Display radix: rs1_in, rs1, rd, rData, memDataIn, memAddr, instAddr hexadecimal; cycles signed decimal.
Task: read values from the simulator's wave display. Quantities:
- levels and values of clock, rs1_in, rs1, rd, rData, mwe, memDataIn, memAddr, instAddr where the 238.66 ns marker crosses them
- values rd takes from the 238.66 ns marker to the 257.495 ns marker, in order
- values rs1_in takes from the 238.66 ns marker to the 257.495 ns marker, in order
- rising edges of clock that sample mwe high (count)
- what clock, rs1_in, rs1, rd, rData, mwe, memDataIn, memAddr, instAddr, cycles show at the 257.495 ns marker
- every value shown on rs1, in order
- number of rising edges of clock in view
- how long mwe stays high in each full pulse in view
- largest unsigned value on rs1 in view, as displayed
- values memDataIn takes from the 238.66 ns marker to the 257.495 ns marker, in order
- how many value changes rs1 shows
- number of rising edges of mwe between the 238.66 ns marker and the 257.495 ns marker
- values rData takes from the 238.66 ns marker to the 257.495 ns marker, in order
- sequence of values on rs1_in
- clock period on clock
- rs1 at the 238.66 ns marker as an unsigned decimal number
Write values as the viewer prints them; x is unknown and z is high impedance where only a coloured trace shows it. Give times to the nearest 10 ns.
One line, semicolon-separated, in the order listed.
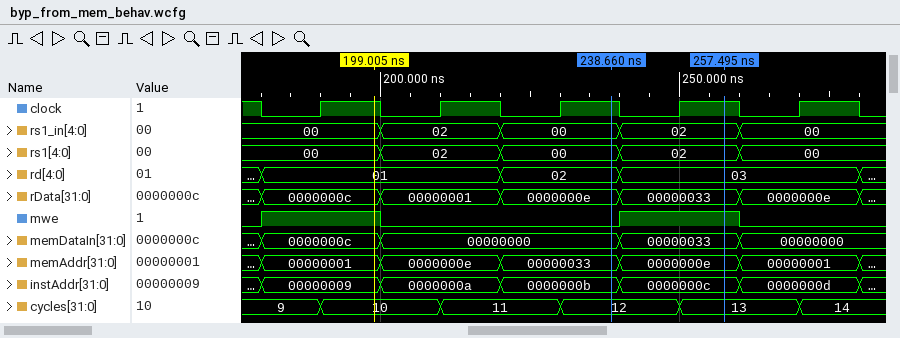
clock=1, rs1_in=00, rs1=00, rd=02, rData=0000000e, mwe=0, memDataIn=00000000, memAddr=00000033, instAddr=0000000b; 02, 03; 00, 02; 2; clock=1, rs1_in=02, rs1=02, rd=03, rData=00000033, mwe=1, memDataIn=00000033, memAddr=0000000e, instAddr=0000000c, cycles=13; 00, 02, 00, 02, 00; 5; 20 ns, 20 ns; 02; 00000000, 00000033; 4; 1; 0000000e, 00000033; 00, 02, 00, 02, 00; 20 ns; 0
